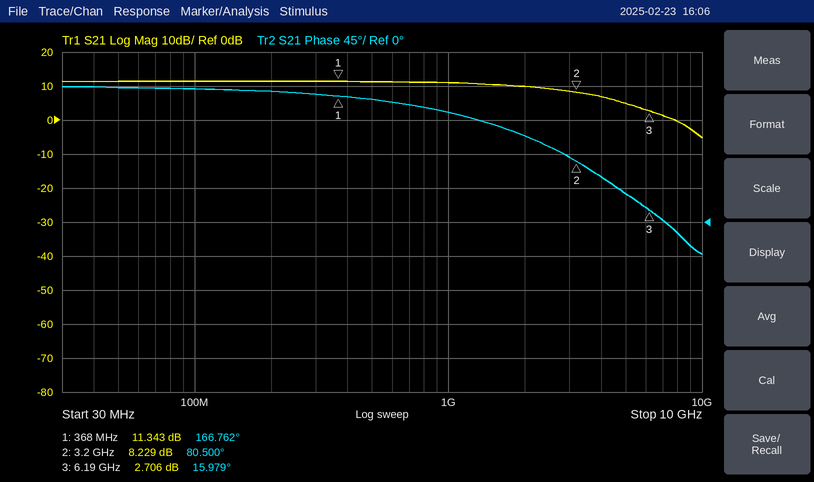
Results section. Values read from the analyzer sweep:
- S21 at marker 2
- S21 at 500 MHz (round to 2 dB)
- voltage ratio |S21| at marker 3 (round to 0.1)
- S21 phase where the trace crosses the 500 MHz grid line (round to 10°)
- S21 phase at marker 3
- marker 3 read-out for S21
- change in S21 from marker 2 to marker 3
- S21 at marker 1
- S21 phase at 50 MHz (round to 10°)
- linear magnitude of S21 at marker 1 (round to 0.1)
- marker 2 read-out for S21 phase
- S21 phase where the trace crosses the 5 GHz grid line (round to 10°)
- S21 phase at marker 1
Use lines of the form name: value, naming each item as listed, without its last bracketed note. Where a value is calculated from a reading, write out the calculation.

S21 at marker 2: 8.229 dB
S21 at 500 MHz: 12 dB
voltage ratio |S21| at marker 3: 10^(2.706/20) ≈ 1.4
S21 phase where the trace crosses the 500 MHz grid line: 160°
S21 phase at marker 3: 15.979°
marker 3 read-out for S21: 2.706 dB
change in S21 from marker 2 to marker 3: 2.706 − (8.229) = -5.523 dB
S21 at marker 1: 11.343 dB
S21 phase at 50 MHz: 180°
linear magnitude of S21 at marker 1: 10^(11.343/20) ≈ 3.7
marker 2 read-out for S21 phase: 80.500°
S21 phase where the trace crosses the 5 GHz grid line: 40°
S21 phase at marker 1: 166.762°
